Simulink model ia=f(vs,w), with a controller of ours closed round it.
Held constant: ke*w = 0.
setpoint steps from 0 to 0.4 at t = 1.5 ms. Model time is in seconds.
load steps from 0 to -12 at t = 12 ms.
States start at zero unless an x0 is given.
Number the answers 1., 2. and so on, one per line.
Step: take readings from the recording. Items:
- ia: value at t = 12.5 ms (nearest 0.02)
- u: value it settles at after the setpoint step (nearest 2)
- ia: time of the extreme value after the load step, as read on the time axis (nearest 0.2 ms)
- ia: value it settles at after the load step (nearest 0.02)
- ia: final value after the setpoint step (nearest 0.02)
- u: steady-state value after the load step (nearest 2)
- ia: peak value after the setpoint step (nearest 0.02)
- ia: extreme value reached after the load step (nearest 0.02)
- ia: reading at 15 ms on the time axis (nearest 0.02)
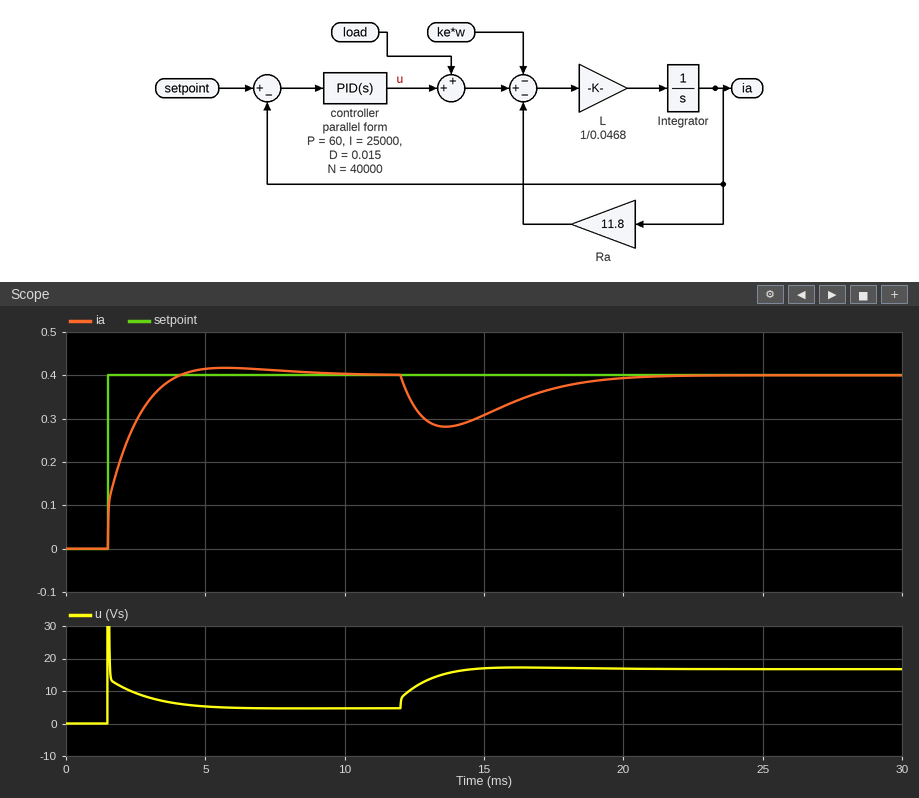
1. 0.32
2. 4
3. 13.6 ms
4. 0.40
5. 0.40
6. 16
7. 0.42
8. 0.28
9. 0.30
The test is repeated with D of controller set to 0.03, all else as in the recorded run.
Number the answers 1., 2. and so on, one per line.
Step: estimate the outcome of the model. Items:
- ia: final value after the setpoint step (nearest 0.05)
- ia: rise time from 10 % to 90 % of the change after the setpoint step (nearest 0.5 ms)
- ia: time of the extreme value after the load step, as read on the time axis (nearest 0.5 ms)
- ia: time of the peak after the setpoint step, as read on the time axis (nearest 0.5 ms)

1. 0.40
2. 2.0 ms
3. 14.0 ms
4. 6.5 ms
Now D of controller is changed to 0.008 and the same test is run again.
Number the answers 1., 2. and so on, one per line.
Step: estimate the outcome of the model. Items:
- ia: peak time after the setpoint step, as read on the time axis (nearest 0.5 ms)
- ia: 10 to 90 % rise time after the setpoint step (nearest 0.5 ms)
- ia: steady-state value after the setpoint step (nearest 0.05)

1. 5.5 ms
2. 1.5 ms
3. 0.40
